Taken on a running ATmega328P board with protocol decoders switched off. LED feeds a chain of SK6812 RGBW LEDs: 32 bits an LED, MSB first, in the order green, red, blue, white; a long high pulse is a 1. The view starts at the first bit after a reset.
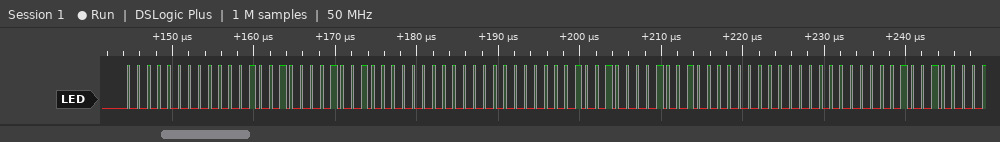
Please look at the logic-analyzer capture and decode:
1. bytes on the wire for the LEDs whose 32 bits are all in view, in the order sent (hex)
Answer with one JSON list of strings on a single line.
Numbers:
["00 09 09 00 00 09 09 00"]
